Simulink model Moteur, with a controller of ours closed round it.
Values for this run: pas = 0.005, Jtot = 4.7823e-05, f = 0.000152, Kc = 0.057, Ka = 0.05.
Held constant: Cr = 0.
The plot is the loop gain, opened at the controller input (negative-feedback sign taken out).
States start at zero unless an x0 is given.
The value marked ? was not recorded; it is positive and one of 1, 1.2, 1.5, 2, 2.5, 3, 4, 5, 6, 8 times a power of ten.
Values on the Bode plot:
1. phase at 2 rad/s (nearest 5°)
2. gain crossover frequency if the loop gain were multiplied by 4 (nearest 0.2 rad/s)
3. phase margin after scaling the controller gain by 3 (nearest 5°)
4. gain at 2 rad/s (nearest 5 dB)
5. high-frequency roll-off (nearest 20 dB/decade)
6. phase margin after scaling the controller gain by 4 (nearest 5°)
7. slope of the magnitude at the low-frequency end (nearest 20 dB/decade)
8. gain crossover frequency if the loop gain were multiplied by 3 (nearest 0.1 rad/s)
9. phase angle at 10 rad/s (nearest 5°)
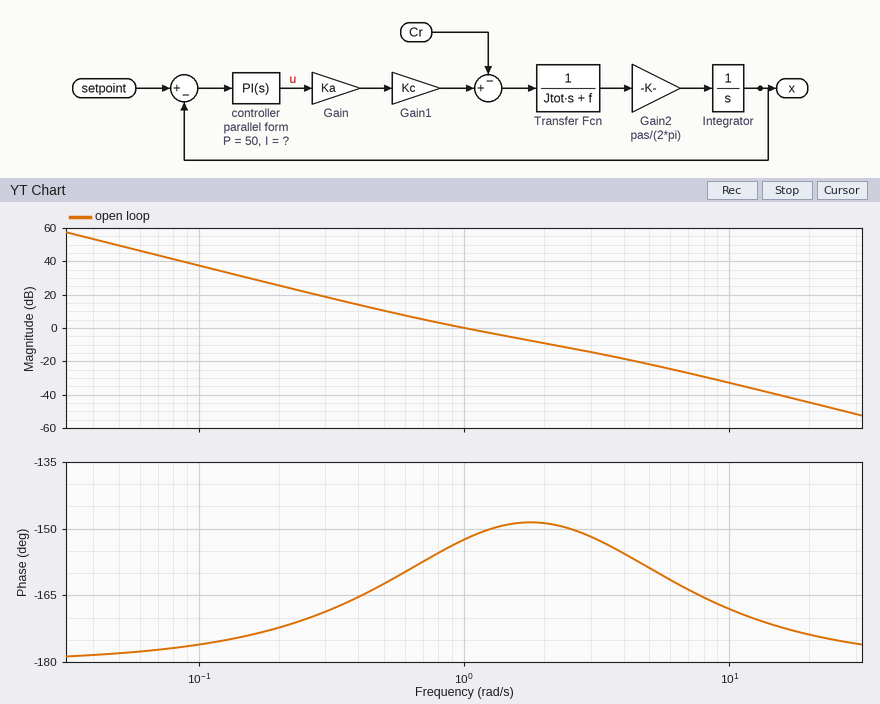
-150°
2.6 rad/s
30°
-10 dB
-40 dB/decade
30°
-40 dB/decade
2.1 rad/s
-170°
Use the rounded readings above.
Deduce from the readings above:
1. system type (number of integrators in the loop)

2
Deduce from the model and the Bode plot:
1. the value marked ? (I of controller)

50
